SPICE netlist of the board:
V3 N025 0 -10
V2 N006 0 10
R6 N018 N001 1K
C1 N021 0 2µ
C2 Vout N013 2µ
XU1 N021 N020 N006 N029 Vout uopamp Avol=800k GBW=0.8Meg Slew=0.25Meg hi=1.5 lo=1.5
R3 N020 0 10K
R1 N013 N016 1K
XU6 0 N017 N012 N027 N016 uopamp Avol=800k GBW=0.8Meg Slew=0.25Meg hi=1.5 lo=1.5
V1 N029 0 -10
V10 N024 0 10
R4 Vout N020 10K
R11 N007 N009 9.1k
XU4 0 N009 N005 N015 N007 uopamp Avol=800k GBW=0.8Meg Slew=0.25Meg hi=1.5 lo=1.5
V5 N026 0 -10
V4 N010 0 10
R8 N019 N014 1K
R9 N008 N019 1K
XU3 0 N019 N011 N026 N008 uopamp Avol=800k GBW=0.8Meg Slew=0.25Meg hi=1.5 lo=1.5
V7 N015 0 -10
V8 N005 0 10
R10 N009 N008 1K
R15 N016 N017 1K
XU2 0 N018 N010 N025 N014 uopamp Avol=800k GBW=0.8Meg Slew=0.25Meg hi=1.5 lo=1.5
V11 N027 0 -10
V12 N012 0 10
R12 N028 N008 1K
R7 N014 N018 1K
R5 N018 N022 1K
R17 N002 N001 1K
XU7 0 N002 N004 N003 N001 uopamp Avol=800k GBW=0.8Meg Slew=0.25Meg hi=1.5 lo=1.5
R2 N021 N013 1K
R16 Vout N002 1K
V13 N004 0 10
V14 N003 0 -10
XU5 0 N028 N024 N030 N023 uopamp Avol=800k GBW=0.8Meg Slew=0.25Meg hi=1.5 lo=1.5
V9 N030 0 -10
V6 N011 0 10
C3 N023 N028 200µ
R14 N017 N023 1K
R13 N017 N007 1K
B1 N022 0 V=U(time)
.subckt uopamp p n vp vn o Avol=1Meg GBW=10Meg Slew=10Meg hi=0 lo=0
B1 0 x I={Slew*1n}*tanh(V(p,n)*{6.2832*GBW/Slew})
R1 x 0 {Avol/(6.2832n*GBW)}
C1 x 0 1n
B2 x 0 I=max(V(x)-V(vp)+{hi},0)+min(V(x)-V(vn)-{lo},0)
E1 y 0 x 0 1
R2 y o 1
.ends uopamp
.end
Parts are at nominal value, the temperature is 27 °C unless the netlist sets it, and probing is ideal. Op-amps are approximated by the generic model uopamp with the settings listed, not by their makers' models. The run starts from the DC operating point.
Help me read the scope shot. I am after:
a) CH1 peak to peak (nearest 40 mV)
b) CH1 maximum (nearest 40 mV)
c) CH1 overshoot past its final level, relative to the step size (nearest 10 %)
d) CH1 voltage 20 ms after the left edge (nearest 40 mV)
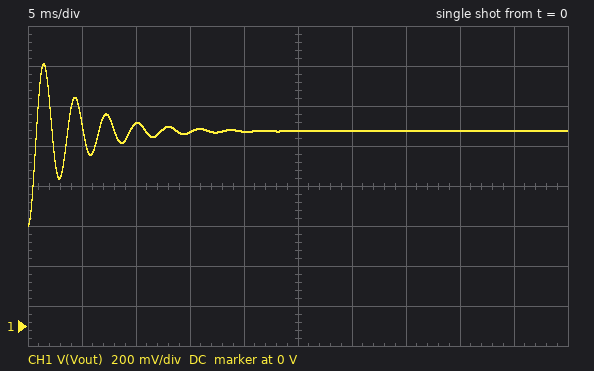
800 mV
1.32 V
70 %
960 mV
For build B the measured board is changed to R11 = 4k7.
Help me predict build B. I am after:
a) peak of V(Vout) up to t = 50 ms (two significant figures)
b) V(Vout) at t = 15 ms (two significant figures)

1.2 V
950 mV
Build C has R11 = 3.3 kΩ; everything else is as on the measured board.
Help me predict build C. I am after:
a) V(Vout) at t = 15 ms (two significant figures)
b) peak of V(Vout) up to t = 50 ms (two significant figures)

930 mV
1.2 V
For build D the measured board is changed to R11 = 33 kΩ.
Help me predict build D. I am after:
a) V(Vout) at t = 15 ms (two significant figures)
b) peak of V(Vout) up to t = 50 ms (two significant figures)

1.0 V
1.4 V
